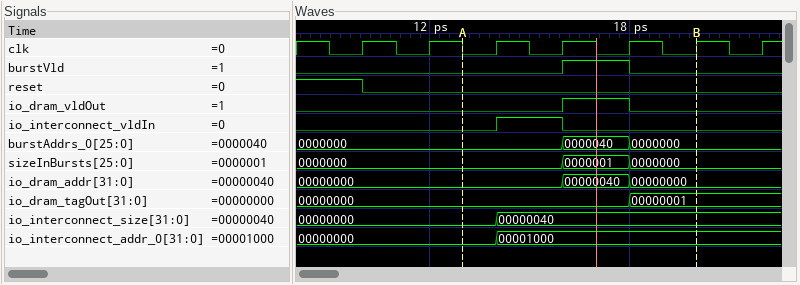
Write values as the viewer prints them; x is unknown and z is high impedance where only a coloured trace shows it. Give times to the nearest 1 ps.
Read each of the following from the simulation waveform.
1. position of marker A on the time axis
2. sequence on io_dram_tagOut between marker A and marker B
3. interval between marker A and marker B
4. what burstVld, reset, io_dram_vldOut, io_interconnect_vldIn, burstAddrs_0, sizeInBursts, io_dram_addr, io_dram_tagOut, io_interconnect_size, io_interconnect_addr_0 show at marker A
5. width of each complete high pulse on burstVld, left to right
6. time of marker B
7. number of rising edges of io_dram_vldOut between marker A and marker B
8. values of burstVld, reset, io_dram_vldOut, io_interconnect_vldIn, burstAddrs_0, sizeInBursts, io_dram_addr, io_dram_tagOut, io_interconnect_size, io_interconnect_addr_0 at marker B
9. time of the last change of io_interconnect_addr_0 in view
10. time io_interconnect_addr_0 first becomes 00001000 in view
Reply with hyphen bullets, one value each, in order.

- 13 ps
- 00000000, 00000001
- 7 ps
- burstVld=0, reset=0, io_dram_vldOut=0, io_interconnect_vldIn=0, burstAddrs_0=0000000, sizeInBursts=0000000, io_dram_addr=00000000, io_dram_tagOut=00000000, io_interconnect_size=00000000, io_interconnect_addr_0=00000000
- 2 ps
- 20 ps
- 1
- burstVld=0, reset=0, io_dram_vldOut=0, io_interconnect_vldIn=0, burstAddrs_0=0000000, sizeInBursts=0000000, io_dram_addr=00000000, io_dram_tagOut=00000001, io_interconnect_size=00000040, io_interconnect_addr_0=00001000
- 14 ps
- 14 ps
